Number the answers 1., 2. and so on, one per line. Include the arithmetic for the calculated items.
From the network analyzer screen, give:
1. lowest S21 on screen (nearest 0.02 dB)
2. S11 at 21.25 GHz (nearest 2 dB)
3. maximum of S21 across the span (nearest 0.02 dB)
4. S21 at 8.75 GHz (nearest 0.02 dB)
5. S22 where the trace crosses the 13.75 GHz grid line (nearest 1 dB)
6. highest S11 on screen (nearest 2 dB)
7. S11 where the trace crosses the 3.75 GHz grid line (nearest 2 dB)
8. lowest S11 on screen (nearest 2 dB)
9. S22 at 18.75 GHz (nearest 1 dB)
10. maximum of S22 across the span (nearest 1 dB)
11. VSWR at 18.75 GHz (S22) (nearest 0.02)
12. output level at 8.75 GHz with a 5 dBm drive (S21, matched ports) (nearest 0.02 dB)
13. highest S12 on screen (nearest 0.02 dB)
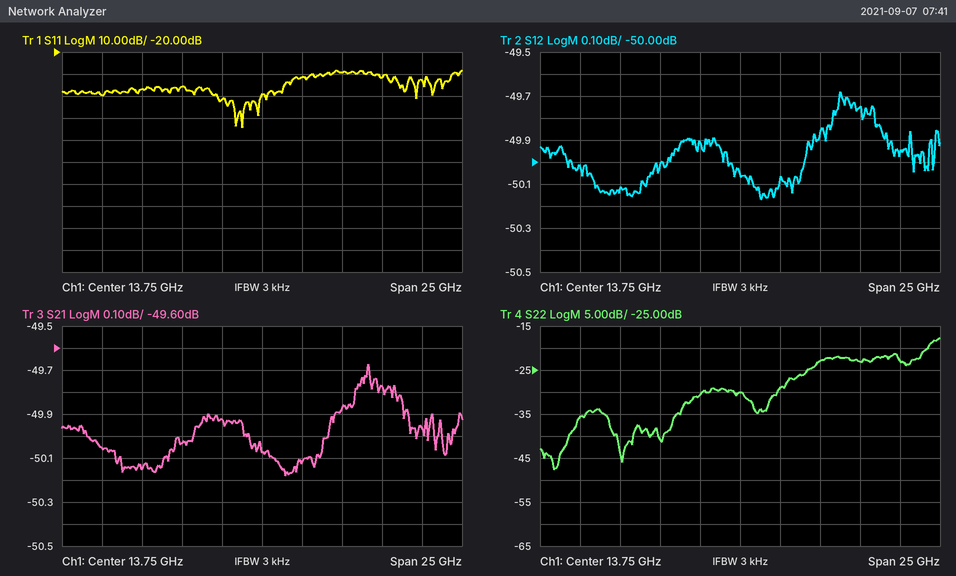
1. -50.18 dB
2. -32 dB
3. -49.68 dB
4. -50.04 dB
5. -30 dB
6. -28 dB
7. -40 dB
8. -54 dB
9. -23 dB
10. -18 dB
11. |Γ| = 10^(-23/20) = 0.0708; VSWR = (1 + 0.0708)/(1 − 0.0708) ≈ 1.15, so 1.16 to the nearest 0.02
12. 5 dBm + (-50.04 dB) = -45.04 dBm
13. -49.68 dB
